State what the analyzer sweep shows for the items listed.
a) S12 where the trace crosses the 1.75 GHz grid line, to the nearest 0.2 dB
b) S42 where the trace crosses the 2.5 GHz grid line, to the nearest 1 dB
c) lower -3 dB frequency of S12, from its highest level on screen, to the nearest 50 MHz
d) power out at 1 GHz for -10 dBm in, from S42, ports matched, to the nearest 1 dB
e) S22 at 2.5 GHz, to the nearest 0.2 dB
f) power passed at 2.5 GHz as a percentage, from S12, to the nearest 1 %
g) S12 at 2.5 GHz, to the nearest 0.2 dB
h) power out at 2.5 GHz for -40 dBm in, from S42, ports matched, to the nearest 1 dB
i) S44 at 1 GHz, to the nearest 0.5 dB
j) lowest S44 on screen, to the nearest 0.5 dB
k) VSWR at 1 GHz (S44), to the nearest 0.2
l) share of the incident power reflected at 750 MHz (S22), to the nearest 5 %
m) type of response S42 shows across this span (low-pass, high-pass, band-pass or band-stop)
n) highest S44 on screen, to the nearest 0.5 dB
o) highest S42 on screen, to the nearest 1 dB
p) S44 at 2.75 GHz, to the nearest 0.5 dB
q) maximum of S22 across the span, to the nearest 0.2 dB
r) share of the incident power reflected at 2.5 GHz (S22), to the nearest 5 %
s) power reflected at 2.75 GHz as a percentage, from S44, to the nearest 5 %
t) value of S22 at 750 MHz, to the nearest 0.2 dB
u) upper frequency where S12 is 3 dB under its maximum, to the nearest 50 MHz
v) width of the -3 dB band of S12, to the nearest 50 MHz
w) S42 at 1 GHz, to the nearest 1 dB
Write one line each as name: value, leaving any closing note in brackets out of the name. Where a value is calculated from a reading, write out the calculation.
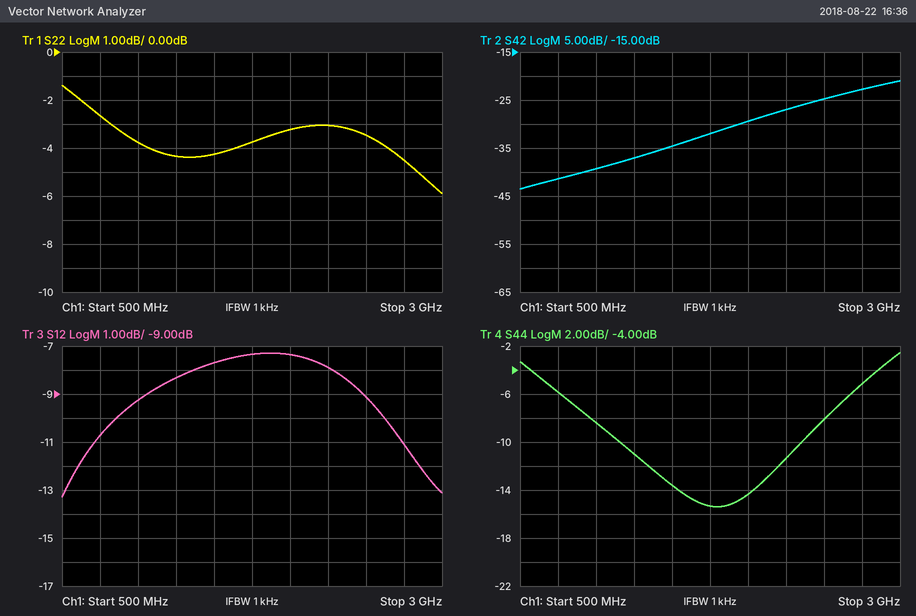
S12 where the trace crosses the 1.75 GHz grid line, to the nearest 0.2 dB: -7.4 dB
S42 where the trace crosses the 2.5 GHz grid line, to the nearest 1 dB: -25 dB
lower -3 dB frequency of S12, from its highest level on screen, to the nearest 50 MHz: 800 MHz
power out at 1 GHz for -10 dBm in, from S42, ports matched, to the nearest 1 dB: -10 dBm + (-39 dB) = -49 dBm
S22 at 2.5 GHz, to the nearest 0.2 dB: -3.4 dB
power passed at 2.5 GHz as a percentage, from S12, to the nearest 1 %: 10^(-9.2/10) ≈ 12 %
S12 at 2.5 GHz, to the nearest 0.2 dB: -9.2 dB
power out at 2.5 GHz for -40 dBm in, from S42, ports matched, to the nearest 1 dB: -40 dBm + (-25 dB) = -65 dBm
S44 at 1 GHz, to the nearest 0.5 dB: -8.5 dB
lowest S44 on screen, to the nearest 0.5 dB: -15.5 dB
VSWR at 1 GHz (S44), to the nearest 0.2: |Γ| = 10^(-8.5/20) = 0.3758; VSWR = (1 + 0.3758)/(1 − 0.3758) ≈ 2.2
share of the incident power reflected at 750 MHz (S22), to the nearest 5 %: 10^(-2.6/10) ≈ 55 %
type of response S42 shows across this span: high-pass
highest S44 on screen, to the nearest 0.5 dB: -2.5 dB
highest S42 on screen, to the nearest 1 dB: -21 dB
S44 at 2.75 GHz, to the nearest 0.5 dB: -5.0 dB
maximum of S22 across the span, to the nearest 0.2 dB: -1.4 dB
share of the incident power reflected at 2.5 GHz (S22), to the nearest 5 %: 10^(-3.4/10) ≈ 45.7 %, so 45 % to the nearest 5 %
power reflected at 2.75 GHz as a percentage, from S44, to the nearest 5 %: 10^(-5/10) ≈ 31.6 %, so 30 % to the nearest 5 %
value of S22 at 750 MHz, to the nearest 0.2 dB: -2.6 dB
upper frequency where S12 is 3 dB under its maximum, to the nearest 50 MHz: 2.65 GHz
width of the -3 dB band of S12, to the nearest 50 MHz: 2.65 GHz − 800 MHz = 1.85 GHz
S42 at 1 GHz, to the nearest 1 dB: -39 dB
